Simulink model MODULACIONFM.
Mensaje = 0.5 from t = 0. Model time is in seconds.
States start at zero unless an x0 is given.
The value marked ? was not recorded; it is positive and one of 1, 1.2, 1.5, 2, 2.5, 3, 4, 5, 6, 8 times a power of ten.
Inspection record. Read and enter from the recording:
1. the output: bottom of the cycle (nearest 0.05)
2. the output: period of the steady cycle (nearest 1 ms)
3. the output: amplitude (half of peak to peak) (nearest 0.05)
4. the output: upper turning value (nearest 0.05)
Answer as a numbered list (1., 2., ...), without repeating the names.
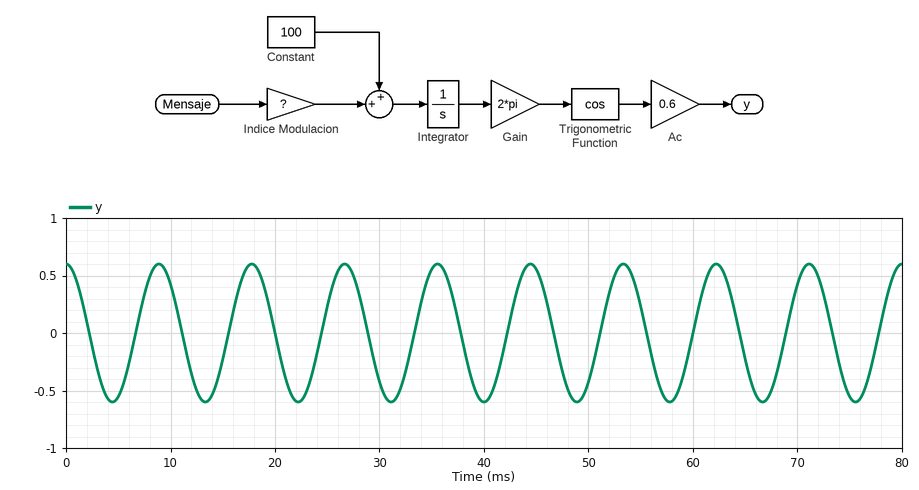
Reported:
1. -0.60
2. 9 ms
3. 0.60
4. 0.60
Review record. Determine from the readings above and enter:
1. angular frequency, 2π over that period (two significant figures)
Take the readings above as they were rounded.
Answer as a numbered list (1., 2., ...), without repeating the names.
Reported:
1. 0.70 rad/ms
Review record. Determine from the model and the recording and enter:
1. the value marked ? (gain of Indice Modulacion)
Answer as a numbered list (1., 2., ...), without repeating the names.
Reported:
1. 25
